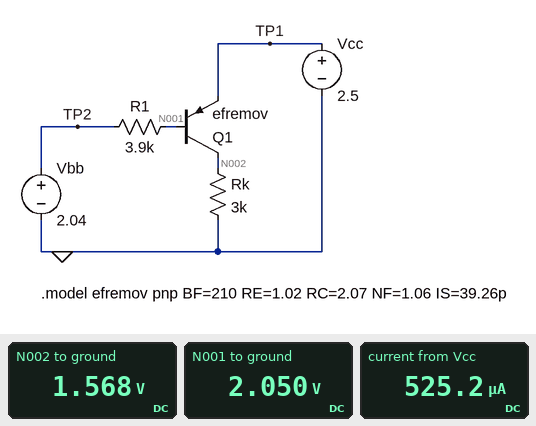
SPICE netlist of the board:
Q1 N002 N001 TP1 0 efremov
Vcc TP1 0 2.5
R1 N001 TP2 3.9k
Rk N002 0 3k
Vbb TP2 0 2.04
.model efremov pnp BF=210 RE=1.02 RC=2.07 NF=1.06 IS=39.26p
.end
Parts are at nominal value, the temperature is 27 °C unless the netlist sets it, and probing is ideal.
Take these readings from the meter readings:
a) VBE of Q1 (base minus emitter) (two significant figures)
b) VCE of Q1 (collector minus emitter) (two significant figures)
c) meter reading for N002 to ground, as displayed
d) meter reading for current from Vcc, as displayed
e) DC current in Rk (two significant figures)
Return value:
-450 mV
-930 mV
1.568 V
525.2 µA
520 µA
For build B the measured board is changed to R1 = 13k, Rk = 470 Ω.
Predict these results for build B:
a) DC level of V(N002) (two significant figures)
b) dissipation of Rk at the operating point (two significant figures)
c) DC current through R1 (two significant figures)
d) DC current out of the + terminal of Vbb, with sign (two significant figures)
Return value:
160 mV
56 µW
1.6 µA
-1.6 µA
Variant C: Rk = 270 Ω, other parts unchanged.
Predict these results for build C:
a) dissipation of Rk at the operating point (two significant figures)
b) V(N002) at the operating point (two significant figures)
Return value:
74 µW
140 mV
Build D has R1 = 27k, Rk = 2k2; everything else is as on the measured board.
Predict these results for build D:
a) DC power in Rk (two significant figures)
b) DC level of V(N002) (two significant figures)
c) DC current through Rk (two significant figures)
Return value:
130 µW
530 mV
240 µA
